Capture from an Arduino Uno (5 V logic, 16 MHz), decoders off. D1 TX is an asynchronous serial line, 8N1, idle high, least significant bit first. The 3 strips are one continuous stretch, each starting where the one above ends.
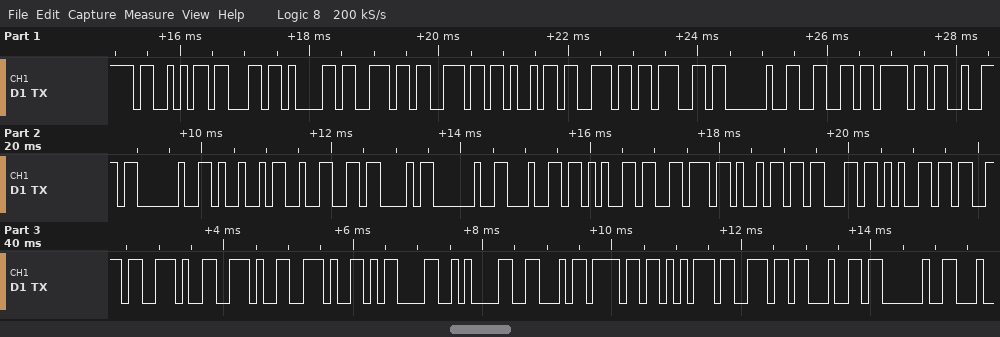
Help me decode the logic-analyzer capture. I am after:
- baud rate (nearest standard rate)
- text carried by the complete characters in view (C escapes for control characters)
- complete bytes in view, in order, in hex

9600 baud
"Scanning for I2C devices...\r\nFound "
53 63 61 6E 6E 69 6E 67 20 66 6F 72 20 49 32 43 20 64 65 76 69 63 65 73 2E 2E 2E 0D 0A 46 6F 75 6E 64 20
